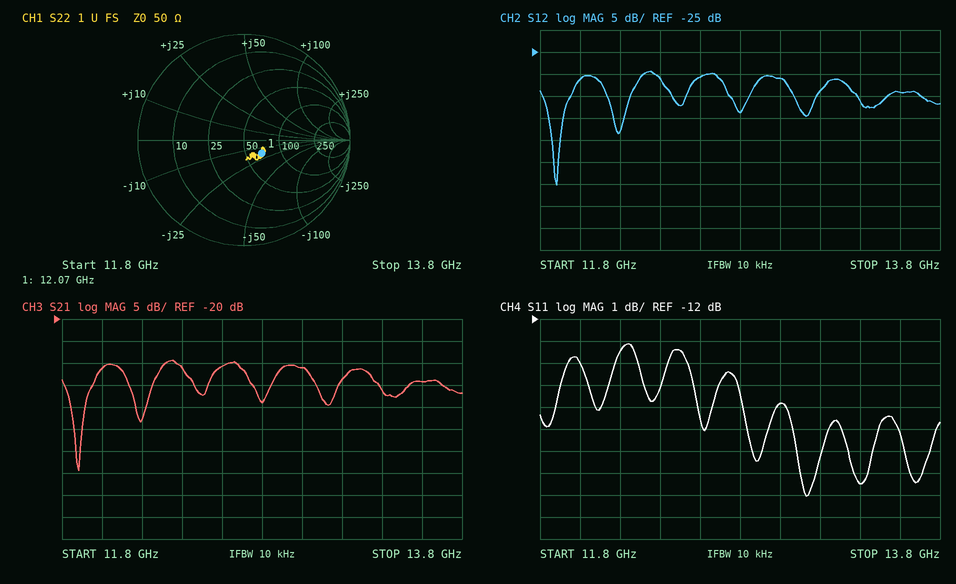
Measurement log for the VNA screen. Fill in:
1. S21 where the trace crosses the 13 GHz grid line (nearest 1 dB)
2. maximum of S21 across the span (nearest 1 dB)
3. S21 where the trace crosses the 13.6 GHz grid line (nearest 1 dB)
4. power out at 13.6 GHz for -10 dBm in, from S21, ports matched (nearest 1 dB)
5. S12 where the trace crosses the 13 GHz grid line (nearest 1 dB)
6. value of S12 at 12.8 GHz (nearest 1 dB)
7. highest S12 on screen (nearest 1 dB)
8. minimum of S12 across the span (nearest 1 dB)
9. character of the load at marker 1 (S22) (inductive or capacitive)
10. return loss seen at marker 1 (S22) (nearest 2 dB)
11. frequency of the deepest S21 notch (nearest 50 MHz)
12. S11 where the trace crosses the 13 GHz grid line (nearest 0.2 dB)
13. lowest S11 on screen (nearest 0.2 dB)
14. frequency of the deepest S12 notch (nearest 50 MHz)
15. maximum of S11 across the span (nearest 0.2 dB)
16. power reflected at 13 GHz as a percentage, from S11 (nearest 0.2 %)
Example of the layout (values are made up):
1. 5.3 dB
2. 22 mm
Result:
1. -31 dB
2. -29 dB
3. -34 dB
4. -44 dBm
5. -31 dB
6. -39 dB
7. -29 dB
8. -55 dB
9. capacitive
10. 14 dB
11. 11.90 GHz
12. -15.8 dB
13. -20.0 dB
14. 11.90 GHz
15. -13.2 dB
16. 2.6 %
